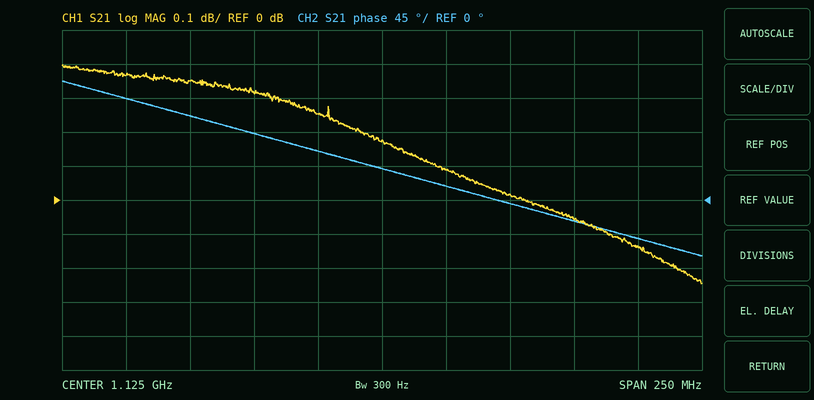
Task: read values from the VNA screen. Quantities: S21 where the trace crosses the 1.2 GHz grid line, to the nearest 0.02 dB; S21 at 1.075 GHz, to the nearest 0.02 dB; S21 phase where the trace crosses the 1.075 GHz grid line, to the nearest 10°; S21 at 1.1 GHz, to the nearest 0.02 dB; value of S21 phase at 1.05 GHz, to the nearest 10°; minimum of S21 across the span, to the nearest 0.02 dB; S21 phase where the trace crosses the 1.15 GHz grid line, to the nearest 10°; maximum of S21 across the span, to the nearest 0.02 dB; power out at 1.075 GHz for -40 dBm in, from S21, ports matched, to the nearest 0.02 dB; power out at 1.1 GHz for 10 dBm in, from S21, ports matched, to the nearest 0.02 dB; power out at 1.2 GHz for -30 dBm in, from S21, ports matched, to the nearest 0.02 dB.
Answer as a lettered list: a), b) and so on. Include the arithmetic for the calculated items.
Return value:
a) -0.06 dB
b) 0.32 dB
c) 90°
d) 0.26 dB
e) 110°
f) -0.24 dB
g) 20°
h) 0.40 dB
i) -40 dBm + (0.32 dB) = -39.68 dBm
j) 10 dBm + (0.26 dB) = 10.26 dBm
k) -30 dBm + (-0.06 dB) = -30.06 dBm
